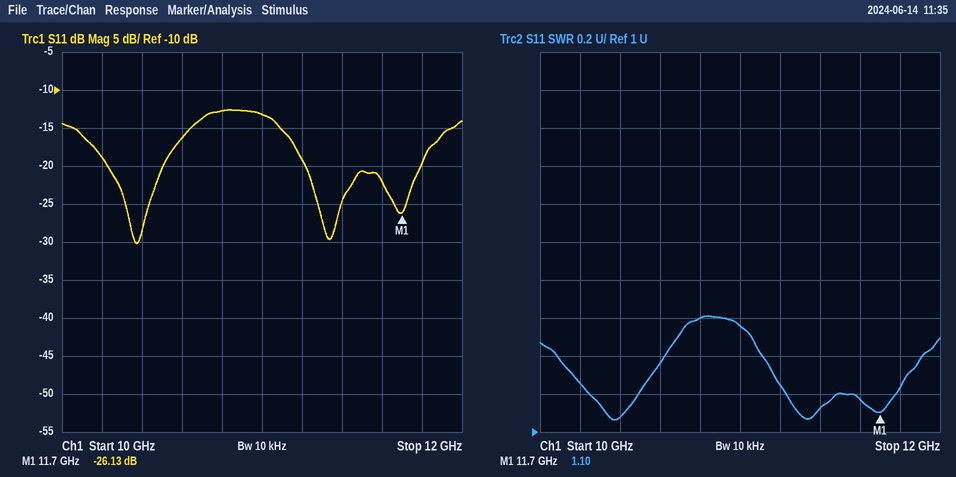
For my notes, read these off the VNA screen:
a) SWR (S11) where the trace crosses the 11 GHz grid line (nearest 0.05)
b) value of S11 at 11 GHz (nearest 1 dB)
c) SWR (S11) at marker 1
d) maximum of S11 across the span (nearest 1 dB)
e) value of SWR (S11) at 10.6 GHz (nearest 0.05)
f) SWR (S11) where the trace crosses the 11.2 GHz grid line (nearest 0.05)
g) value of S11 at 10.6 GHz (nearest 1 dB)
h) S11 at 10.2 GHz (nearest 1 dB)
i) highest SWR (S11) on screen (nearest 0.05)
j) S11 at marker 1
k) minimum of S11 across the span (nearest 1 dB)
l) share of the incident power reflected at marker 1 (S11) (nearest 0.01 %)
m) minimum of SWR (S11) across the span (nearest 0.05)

1.55
-13 dB
1.10
-13 dB
1.35
1.25
-16 dB
-19 dB
1.60
-26.13 dB
-30 dB
0.24 %
1.05
